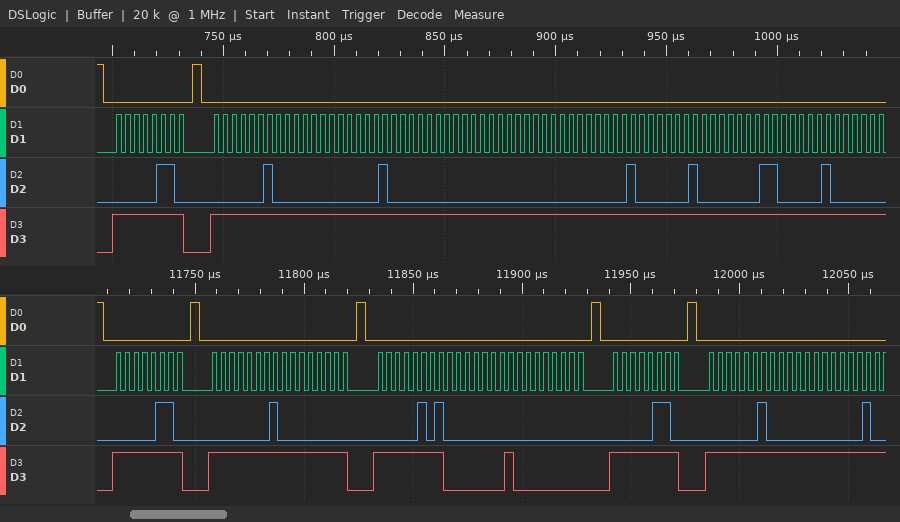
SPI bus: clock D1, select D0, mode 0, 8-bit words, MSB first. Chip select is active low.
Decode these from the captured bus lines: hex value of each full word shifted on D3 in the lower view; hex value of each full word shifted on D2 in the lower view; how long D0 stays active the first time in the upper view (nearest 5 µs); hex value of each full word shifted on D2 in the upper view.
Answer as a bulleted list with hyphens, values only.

- FF, FF, FF, FF, 01, 00, FF, FF, FF
- 06, 01, 00, 05, 00, 00, 06, 02, 00
- 40 µs
- 06, 02, 00, 10, 00, 00, 01, 02, 03, 04
